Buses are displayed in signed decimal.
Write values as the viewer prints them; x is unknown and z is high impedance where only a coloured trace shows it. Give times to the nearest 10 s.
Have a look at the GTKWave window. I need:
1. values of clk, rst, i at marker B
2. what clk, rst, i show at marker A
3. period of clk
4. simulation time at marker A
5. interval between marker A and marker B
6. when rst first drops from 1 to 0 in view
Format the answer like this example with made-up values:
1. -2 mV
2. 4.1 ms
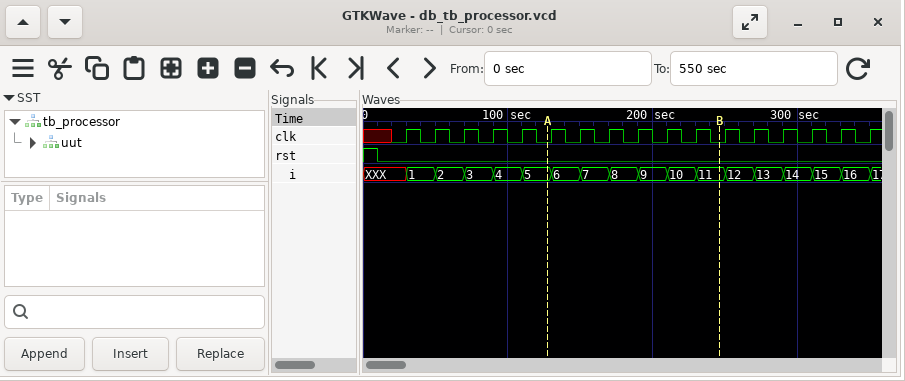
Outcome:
1. clk=0, rst=0, i=11
2. clk=0, rst=0, i=5
3. 20 s
4. 130 s
5. 120 s
6. 10 s
